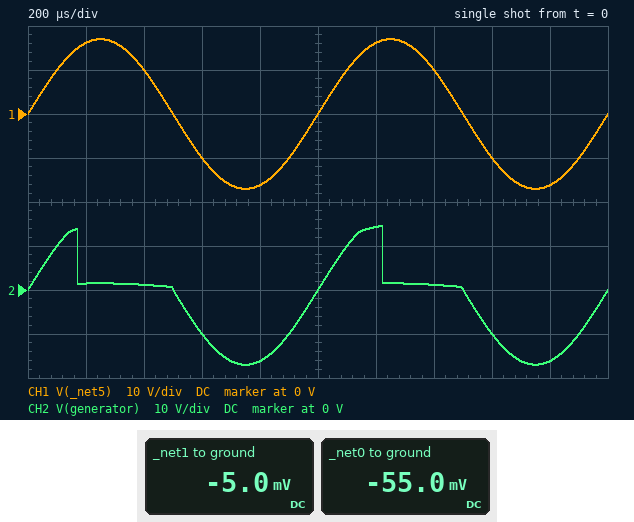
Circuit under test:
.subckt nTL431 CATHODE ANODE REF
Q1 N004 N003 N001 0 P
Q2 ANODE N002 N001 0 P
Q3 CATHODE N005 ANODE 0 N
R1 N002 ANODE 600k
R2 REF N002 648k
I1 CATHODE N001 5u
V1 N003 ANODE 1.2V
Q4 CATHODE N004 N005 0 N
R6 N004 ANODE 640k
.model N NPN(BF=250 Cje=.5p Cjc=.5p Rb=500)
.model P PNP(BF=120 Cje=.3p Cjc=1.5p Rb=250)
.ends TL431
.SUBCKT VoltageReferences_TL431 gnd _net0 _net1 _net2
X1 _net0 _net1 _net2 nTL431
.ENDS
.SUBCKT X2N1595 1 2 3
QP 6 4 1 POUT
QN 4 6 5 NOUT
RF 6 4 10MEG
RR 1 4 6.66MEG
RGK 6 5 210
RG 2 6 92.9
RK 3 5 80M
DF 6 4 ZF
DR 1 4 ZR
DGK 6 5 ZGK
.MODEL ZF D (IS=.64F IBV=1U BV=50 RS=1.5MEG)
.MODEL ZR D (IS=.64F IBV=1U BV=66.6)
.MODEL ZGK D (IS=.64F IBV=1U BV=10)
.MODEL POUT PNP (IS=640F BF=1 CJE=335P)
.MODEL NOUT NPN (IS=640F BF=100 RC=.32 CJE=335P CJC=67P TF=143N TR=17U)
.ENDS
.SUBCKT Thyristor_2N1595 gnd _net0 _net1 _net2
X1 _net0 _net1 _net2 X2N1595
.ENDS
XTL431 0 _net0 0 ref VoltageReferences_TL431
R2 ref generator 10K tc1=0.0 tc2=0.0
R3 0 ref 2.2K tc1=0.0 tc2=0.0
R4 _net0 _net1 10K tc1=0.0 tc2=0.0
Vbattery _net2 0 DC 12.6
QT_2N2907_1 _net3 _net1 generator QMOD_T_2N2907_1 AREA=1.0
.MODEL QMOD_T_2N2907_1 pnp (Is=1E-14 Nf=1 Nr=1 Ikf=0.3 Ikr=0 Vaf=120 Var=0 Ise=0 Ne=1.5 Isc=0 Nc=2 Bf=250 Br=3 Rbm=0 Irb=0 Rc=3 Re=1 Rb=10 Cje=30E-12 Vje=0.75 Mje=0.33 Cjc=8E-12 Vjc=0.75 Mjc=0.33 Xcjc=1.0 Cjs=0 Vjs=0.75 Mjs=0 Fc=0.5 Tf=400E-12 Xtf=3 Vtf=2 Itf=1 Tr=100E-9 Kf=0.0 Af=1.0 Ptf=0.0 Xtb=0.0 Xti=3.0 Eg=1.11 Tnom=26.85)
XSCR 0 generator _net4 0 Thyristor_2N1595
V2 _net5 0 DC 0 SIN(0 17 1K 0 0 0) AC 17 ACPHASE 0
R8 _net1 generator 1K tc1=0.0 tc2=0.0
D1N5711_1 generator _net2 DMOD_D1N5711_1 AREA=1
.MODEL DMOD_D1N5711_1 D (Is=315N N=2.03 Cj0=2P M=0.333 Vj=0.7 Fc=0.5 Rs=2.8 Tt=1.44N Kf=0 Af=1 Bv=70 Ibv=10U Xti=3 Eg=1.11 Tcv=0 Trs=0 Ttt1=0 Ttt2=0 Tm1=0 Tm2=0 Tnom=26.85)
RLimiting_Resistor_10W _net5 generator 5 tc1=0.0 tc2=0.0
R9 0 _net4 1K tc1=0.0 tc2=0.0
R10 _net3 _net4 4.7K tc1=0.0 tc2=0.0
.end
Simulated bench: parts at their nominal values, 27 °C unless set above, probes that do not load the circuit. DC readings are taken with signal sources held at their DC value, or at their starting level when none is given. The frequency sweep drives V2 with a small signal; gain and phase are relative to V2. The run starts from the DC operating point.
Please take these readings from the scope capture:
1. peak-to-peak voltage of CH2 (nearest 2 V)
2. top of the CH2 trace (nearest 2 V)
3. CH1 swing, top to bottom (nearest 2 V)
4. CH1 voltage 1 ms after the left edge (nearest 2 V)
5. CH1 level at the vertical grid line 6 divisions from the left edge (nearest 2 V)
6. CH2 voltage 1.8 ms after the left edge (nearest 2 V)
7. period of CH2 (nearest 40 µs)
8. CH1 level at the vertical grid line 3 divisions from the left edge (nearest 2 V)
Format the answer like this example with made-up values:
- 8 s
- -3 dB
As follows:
- 32 V
- 14 V
- 34 V
- 0 V
- 16 V
- -16 V
- 1.00 ms
- -10 V
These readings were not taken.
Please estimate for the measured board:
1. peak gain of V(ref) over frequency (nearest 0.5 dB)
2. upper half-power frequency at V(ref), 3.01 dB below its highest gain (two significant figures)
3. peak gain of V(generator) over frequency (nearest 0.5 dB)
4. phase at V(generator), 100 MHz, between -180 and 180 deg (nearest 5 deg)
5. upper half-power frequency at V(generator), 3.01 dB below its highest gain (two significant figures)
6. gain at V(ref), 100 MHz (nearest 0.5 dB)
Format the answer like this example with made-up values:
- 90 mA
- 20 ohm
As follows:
- -15.0 dB
- 610 MHz
- 0 dB
- -10 deg
- 610 MHz
- -15.0 dB
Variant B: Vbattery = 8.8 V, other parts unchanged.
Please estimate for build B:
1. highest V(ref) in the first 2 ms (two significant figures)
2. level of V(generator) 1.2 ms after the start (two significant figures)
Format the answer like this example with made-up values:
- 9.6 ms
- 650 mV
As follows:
- 2.2 V
- 12 V
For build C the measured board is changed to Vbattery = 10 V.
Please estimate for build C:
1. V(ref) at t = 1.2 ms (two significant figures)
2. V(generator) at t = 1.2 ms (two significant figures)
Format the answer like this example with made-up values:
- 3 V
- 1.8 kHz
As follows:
- 2.3 V
- 13 V
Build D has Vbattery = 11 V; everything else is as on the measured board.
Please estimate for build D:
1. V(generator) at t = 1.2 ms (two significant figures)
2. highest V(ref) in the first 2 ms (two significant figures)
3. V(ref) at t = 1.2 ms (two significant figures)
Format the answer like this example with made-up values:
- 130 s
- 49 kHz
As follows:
- 13 V
- 2.5 V
- 2.4 V
